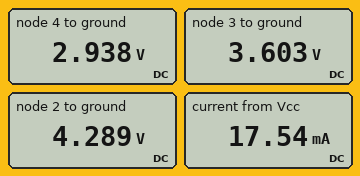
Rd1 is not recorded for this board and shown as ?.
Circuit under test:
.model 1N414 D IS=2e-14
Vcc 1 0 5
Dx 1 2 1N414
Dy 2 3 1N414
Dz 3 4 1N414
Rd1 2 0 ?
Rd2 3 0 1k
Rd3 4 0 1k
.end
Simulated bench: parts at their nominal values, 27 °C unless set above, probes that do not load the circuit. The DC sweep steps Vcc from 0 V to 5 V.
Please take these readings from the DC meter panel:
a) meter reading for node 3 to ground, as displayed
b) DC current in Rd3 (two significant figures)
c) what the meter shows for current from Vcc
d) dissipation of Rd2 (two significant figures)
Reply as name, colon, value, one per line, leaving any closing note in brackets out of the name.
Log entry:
meter reading for node 3 to ground, as displayed: 3.603 V
DC current in Rd3: 2.9 mA
what the meter shows for current from Vcc: 17.54 mA
dissipation of Rd2: 13 mW
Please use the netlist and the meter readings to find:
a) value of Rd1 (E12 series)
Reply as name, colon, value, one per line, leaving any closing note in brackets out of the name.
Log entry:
value of Rd1: 390 Ω
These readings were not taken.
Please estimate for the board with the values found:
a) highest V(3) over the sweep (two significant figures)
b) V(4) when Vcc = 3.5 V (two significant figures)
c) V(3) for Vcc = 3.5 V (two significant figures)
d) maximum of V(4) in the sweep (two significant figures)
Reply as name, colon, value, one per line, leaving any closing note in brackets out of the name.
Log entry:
highest V(3) over the sweep: 3.6 V
V(4) when Vcc = 3.5 V: 1.5 V
V(3) for Vcc = 3.5 V: 2.1 V
maximum of V(4) in the sweep: 2.9 V
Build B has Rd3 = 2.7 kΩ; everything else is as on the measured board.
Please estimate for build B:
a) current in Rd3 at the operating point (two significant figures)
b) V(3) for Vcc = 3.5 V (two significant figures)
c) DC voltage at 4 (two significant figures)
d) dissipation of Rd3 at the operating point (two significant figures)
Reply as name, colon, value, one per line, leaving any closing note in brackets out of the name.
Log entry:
current in Rd3 at the operating point: 1.1 mA
V(3) for Vcc = 3.5 V: 2.1 V
DC voltage at 4: 3.0 V
dissipation of Rd3 at the operating point: 3.3 mW
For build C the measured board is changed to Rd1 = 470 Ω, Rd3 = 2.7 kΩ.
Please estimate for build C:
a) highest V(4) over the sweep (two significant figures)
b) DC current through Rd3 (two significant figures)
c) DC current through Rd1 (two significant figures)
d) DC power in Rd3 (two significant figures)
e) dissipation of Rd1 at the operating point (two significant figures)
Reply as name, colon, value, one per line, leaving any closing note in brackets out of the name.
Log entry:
highest V(4) over the sweep: 3.0 V
DC current through Rd3: 1.1 mA
DC current through Rd1: 9.1 mA
DC power in Rd3: 3.3 mW
dissipation of Rd1 at the operating point: 39 mW
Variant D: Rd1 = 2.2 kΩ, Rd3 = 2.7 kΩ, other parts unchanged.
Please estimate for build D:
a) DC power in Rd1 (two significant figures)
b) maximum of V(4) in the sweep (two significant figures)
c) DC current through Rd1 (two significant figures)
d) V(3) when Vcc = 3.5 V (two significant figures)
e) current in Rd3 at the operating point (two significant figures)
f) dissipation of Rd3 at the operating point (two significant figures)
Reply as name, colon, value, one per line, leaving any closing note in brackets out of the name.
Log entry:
DC power in Rd1: 8.5 mW
maximum of V(4) in the sweep: 3.0 V
DC current through Rd1: 2.0 mA
V(3) when Vcc = 3.5 V: 2.2 V
current in Rd3 at the operating point: 1.1 mA
dissipation of Rd3 at the operating point: 3.3 mW
